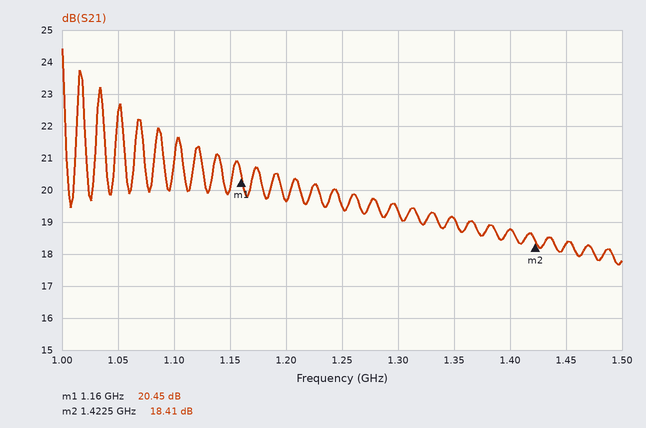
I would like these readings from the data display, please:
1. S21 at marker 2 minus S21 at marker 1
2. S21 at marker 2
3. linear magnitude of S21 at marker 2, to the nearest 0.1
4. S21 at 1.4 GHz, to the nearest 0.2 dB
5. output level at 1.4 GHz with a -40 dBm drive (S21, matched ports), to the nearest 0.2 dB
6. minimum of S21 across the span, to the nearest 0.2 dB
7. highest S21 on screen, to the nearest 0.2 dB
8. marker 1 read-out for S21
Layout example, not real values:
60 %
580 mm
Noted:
-2.04 dB
18.41 dB
8.3
18.8 dB
-21.2 dBm
17.6 dB
24.4 dB
20.45 dB
